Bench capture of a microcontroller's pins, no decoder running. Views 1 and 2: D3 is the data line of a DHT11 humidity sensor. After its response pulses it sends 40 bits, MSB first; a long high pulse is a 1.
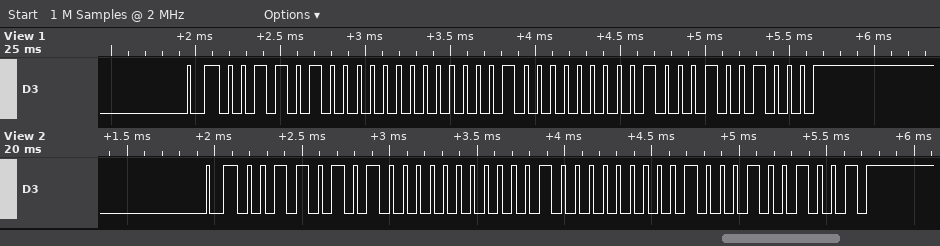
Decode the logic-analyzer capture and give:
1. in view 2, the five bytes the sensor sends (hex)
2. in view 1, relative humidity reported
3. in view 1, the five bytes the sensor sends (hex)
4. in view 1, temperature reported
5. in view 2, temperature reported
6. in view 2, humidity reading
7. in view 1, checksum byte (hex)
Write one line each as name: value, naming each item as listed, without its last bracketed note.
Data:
in view 2, the five bytes the sensor sends: 35 00 10 04 49
in view 1, relative humidity reported: 52 %
in view 1, the five bytes the sensor sends: 34 00 10 04 48
in view 1, temperature reported: 16.4 °C
in view 2, temperature reported: 16.4 °C
in view 2, humidity reading: 53 %
in view 1, checksum byte: 0x48
